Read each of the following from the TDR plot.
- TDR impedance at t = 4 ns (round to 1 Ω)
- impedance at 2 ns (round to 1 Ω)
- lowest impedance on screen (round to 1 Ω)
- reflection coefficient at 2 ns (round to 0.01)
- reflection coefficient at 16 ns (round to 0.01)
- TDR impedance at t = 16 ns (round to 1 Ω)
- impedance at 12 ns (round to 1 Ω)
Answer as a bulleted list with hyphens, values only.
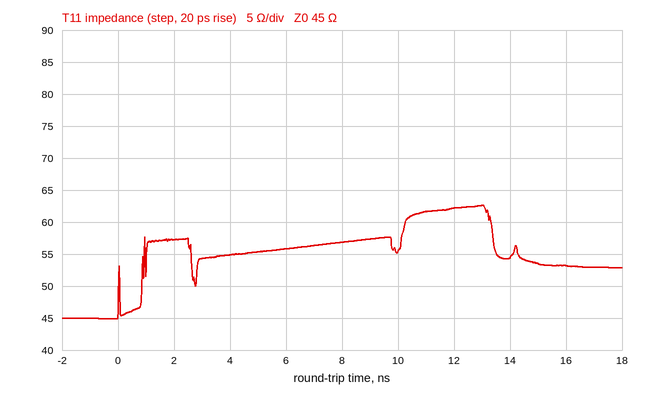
- 55 Ω
- 57 Ω
- 45 Ω
- +0.12
- +0.08
- 53 Ω
- 62 Ω
